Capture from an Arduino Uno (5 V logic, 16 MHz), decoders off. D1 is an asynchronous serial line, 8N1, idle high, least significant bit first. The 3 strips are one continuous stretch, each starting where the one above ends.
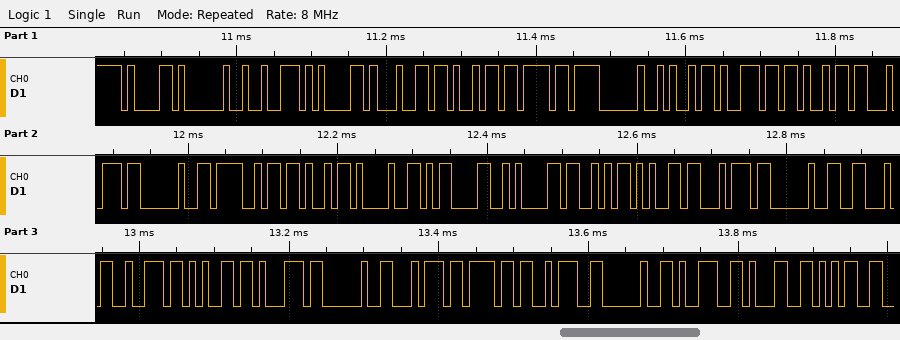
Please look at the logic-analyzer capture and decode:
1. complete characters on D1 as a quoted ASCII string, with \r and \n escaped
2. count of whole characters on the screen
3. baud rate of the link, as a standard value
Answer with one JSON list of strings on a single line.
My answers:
["\"a radio init OK!\\r\\nSet Freq to: 915\"", "34", "115200 baud"]
